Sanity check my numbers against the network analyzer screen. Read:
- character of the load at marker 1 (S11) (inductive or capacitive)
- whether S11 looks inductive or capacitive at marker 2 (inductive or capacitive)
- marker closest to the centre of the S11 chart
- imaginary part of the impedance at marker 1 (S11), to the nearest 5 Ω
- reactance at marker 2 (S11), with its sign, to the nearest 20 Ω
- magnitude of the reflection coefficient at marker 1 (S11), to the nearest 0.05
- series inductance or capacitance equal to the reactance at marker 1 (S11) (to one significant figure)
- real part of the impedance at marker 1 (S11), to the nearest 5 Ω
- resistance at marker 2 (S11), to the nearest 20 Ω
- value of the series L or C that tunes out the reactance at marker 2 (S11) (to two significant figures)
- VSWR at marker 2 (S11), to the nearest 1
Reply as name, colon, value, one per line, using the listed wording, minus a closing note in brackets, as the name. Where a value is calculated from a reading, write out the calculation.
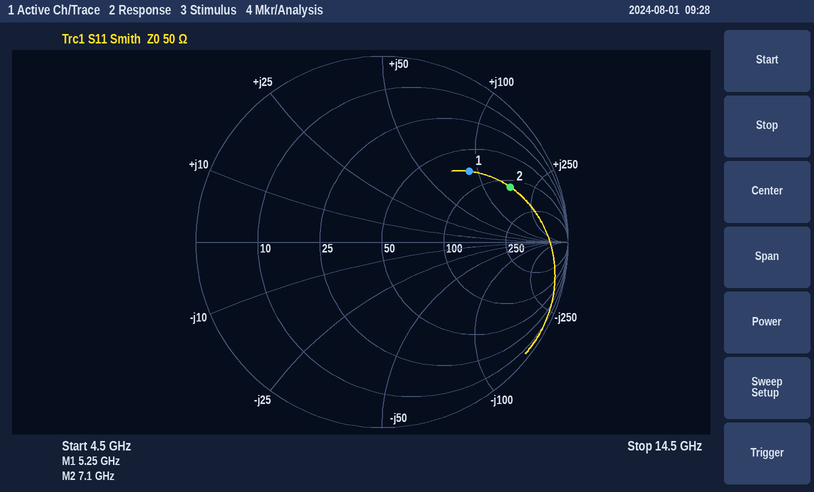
character of the load at marker 1 (S11): inductive
whether S11 looks inductive or capacitive at marker 2: inductive
marker closest to the centre of the S11 chart: marker 1
imaginary part of the impedance at marker 1 (S11), to the nearest 5 Ω: +90 Ω
reactance at marker 2 (S11), with its sign, to the nearest 20 Ω: +160 Ω
magnitude of the reflection coefficient at marker 1 (S11), to the nearest 0.05: 0.60
series inductance or capacitance equal to the reactance at marker 1 (S11): L = 90 Ω/(2π × 5.25 GHz) ≈ 3 nH
real part of the impedance at marker 1 (S11), to the nearest 5 Ω: 75 Ω
resistance at marker 2 (S11), to the nearest 20 Ω: 120 Ω
value of the series L or C that tunes out the reactance at marker 2 (S11): C = 1/(2π × 7.1 GHz × 160 Ω) ≈ 140 fF
VSWR at marker 2 (S11), to the nearest 1: 7
